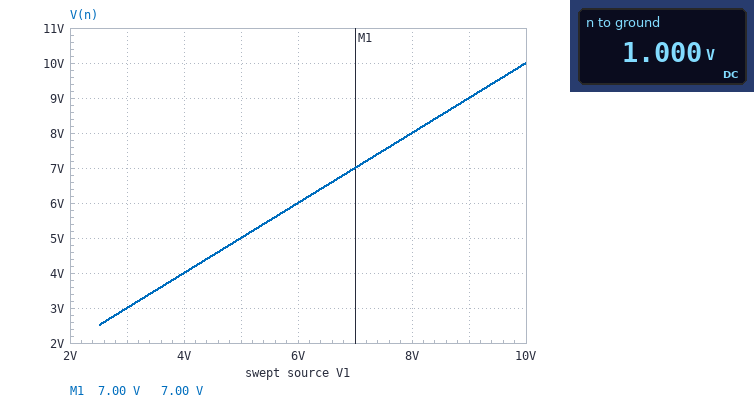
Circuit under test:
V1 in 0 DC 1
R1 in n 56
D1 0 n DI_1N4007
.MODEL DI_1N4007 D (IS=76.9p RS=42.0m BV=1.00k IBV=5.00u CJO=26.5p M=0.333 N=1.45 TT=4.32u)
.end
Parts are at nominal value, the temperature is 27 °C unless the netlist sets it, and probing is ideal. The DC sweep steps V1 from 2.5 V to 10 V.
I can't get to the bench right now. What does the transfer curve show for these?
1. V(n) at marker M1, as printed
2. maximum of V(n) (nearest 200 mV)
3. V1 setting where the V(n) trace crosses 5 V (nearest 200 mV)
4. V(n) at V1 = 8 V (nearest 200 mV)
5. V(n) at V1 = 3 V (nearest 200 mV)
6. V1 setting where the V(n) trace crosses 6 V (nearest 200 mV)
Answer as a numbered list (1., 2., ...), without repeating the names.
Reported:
1. 7.00 V
2. 10.0 V
3. 5.0 V
4. 8.0 V
5. 3.0 V
6. 6.0 V
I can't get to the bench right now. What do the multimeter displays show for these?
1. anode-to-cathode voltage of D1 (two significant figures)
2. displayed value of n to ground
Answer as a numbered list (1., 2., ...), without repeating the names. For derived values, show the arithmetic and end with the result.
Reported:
1. 0 V - 1 V = -1.0 V
2. 1.000 V
